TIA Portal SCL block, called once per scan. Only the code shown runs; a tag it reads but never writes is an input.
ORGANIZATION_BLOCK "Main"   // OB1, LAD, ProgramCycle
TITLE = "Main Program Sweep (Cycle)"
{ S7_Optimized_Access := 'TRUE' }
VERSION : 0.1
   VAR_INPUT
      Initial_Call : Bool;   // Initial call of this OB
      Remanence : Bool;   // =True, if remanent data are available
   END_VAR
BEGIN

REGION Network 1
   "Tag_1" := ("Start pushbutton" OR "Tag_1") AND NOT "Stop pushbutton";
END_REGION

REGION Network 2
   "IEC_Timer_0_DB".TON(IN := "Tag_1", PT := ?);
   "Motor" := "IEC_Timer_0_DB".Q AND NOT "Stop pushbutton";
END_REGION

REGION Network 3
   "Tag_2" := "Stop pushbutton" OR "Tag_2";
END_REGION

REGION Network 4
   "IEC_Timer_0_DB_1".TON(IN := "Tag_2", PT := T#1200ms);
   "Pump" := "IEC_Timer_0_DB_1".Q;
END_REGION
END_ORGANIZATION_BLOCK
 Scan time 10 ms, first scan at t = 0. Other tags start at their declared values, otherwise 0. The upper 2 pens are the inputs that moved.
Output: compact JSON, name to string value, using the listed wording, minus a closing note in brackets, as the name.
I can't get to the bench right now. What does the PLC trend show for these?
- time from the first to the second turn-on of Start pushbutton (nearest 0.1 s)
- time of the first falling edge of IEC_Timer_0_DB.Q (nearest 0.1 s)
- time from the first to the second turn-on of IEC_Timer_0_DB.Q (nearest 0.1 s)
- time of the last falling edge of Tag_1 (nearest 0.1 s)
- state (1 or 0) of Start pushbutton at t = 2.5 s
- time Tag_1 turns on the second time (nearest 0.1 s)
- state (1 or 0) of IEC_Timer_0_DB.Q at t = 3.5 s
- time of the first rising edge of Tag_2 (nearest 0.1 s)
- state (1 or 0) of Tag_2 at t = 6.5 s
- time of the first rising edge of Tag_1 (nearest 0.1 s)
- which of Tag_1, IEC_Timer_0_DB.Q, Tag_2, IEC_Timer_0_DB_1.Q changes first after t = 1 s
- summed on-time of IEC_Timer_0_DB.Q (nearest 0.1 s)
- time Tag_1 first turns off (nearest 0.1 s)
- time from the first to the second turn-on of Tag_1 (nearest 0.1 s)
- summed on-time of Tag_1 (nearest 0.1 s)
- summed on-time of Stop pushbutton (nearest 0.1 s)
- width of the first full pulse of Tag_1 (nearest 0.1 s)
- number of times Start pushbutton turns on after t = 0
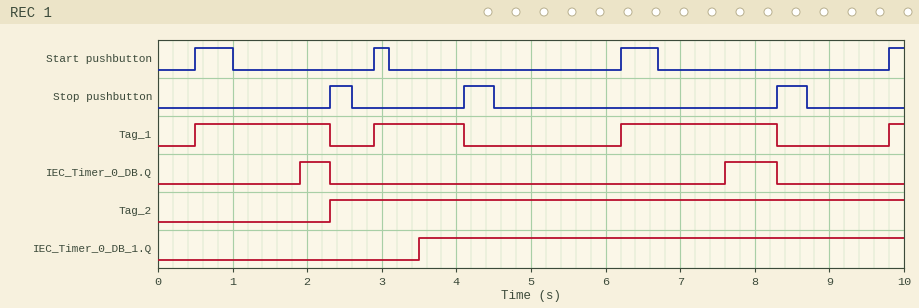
{"time from the first to the second turn-on of Start pushbutton": "2.4 s", "time of the first falling edge of IEC_Timer_0_DB.Q": "2.3 s", "time from the first to the second turn-on of IEC_Timer_0_DB.Q": "5.7 s", "time of the last falling edge of Tag_1": "8.3 s", "state (1 or 0) of Start pushbutton at t = 2.5 s": "0", "time Tag_1 turns on the second time": "2.9 s", "state (1 or 0) of IEC_Timer_0_DB.Q at t = 3.5 s": "0", "time of the first rising edge of Tag_2": "2.3 s", "state (1 or 0) of Tag_2 at t = 6.5 s": "1", "time of the first rising edge of Tag_1": "0.5 s", "which of Tag_1, IEC_Timer_0_DB.Q, Tag_2, IEC_Timer_0_DB_1.Q changes first after t = 1 s": "IEC_Timer_0_DB.Q", "summed on-time of IEC_Timer_0_DB.Q": "1.1 s", "time Tag_1 first turns off": "2.3 s", "time from the first to the second turn-on of Tag_1": "2.4 s", "summed on-time of Tag_1": "5.3 s", "summed on-time of Stop pushbutton": "1.1 s", "width of the first full pulse of Tag_1": "1.8 s", "number of times Start pushbutton turns on after t = 0": "4"}
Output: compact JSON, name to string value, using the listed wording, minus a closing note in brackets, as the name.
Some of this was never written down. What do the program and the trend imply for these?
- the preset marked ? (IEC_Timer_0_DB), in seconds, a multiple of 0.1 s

{"the preset marked ? (IEC_Timer_0_DB), in seconds, a multiple of 0.1 s": "1.4 s"}
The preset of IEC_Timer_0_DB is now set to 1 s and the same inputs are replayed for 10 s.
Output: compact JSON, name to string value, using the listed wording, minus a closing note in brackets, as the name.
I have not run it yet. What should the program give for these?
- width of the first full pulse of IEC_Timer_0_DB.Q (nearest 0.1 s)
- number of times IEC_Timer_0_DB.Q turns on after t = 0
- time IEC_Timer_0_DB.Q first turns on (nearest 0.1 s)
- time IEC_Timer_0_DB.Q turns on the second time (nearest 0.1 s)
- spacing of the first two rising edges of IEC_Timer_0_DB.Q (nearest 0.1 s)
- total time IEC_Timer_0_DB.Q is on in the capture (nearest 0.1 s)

{"width of the first full pulse of IEC_Timer_0_DB.Q": "0.8 s", "number of times IEC_Timer_0_DB.Q turns on after t = 0": "3", "time IEC_Timer_0_DB.Q first turns on": "1.5 s", "time IEC_Timer_0_DB.Q turns on the second time": "3.9 s", "spacing of the first two rising edges of IEC_Timer_0_DB.Q": "2.4 s", "total time IEC_Timer_0_DB.Q is on in the capture": "2.1 s"}
